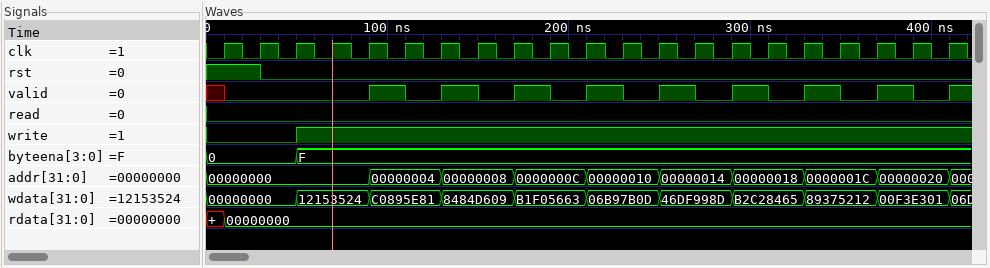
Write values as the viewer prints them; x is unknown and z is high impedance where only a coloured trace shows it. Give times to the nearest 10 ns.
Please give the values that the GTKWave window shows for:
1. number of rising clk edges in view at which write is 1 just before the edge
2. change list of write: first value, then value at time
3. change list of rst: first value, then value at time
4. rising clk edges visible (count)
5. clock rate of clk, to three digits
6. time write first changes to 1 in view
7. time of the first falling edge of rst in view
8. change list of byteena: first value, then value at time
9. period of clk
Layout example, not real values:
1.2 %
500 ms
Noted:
18
0, 1 at 50 ns
1, 0 at 30 ns
21
50.0 MHz
50 ns
30 ns
0, F at 50 ns
20 ns
